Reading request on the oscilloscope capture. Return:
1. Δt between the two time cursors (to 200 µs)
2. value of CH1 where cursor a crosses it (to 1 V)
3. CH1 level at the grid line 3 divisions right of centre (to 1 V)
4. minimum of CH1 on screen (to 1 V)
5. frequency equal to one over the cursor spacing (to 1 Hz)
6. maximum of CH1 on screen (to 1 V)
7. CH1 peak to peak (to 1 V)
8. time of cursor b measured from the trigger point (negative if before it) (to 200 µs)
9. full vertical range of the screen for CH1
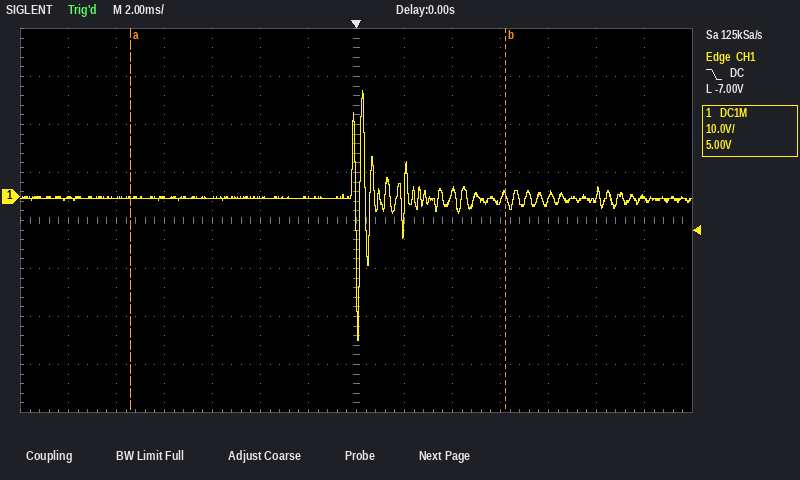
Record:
15.6 ms
0 V
-1 V
-30 V
64 Hz
22 V
52 V
+6.2 ms
80 V
